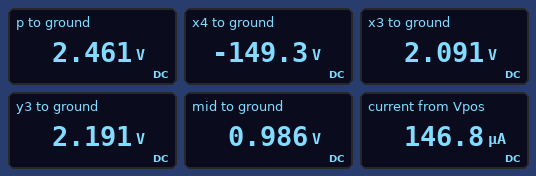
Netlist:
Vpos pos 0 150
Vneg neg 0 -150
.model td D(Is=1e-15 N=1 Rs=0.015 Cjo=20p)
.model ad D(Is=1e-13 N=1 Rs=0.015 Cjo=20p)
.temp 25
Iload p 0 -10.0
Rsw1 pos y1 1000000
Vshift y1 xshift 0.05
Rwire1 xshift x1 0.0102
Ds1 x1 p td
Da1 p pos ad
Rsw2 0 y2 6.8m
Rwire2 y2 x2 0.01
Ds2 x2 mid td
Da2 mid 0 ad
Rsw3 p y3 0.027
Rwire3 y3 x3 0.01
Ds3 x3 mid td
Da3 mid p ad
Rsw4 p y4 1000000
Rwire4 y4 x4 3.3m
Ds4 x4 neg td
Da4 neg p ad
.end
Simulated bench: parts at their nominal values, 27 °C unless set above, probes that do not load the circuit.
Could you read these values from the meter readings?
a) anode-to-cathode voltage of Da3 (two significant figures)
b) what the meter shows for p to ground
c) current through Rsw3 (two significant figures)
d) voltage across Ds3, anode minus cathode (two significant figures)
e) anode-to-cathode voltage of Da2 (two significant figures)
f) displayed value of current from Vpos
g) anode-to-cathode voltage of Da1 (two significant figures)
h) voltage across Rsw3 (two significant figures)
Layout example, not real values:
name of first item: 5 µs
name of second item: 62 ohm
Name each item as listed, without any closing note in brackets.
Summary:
anode-to-cathode voltage of Da3: -1.5 V
what the meter shows for p to ground: 2.461 V
current through Rsw3: 10 A
voltage across Ds3, anode minus cathode: 1.1 V
anode-to-cathode voltage of Da2: 990 mV
displayed value of current from Vpos: 146.8 µA
anode-to-cathode voltage of Da1: -150 V
voltage across Rsw3: 270 mV
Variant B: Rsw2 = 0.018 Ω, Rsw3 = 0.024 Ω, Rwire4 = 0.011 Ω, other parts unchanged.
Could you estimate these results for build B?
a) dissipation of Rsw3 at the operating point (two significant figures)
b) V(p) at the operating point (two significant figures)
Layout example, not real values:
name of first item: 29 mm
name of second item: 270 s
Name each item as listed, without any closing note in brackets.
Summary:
dissipation of Rsw3 at the operating point: 2.4 W
V(p) at the operating point: 2.4 V
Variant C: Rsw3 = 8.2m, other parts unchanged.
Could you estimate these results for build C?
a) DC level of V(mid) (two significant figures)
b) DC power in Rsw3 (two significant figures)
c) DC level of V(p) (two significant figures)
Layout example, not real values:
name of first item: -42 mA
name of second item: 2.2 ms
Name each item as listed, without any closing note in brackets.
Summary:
DC level of V(mid): 990 mV
DC power in Rsw3: 820 mW
DC level of V(p): 2.3 V
